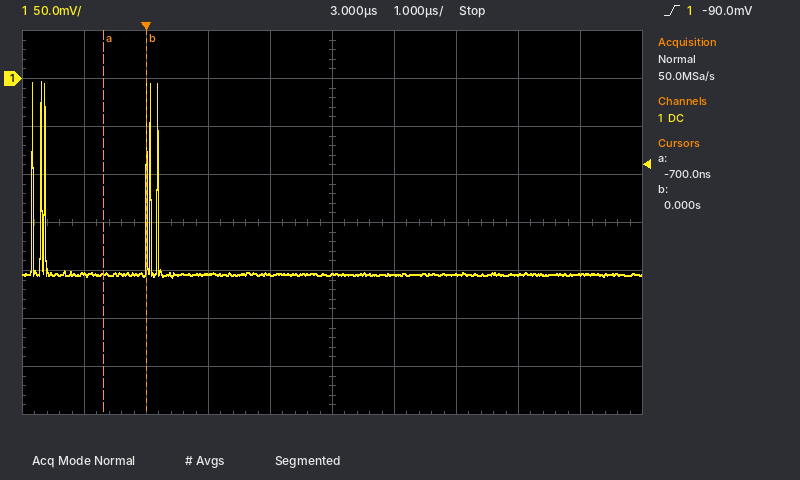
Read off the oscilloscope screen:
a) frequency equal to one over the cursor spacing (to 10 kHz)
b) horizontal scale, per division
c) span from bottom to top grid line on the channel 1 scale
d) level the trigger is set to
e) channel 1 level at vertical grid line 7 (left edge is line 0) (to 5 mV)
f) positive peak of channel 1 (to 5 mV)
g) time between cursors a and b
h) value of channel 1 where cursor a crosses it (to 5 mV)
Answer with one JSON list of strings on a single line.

["1.43 MHz", "1 µs", "400 mV", "-90.0 mV", "-205 mV", "-5 mV", "700 ns", "-205 mV"]
